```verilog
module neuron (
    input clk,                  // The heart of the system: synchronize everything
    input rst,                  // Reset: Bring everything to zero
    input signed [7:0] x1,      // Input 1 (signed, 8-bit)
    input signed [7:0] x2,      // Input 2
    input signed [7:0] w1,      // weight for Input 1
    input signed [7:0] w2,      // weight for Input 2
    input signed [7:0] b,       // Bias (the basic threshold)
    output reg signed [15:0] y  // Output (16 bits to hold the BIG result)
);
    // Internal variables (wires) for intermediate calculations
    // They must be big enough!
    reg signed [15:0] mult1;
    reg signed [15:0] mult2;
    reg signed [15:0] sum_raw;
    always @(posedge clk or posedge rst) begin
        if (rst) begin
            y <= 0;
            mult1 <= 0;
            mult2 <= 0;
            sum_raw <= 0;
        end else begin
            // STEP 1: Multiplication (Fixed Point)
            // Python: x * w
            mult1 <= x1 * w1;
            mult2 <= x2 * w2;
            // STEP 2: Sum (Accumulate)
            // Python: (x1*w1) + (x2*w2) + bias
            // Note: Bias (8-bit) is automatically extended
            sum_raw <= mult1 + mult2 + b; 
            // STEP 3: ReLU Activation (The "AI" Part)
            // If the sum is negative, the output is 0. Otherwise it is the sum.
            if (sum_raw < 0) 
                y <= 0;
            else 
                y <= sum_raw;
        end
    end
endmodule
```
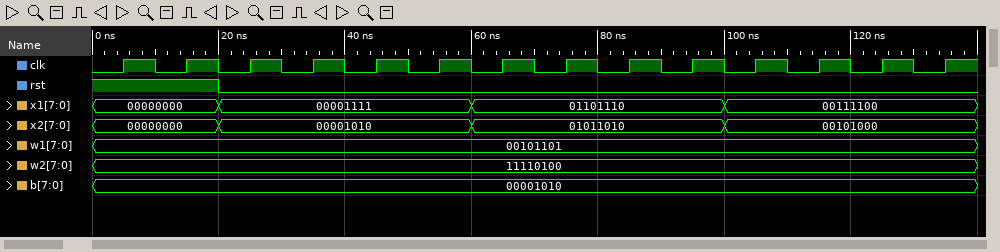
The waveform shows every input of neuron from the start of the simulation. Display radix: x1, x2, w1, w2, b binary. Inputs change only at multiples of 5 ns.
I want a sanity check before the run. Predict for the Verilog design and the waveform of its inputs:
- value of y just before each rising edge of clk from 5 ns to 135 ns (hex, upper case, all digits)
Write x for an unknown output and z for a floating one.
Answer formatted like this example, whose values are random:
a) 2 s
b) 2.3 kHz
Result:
a) 0000, 0000, 0000, 0000, 000A, 0235, 0235, 0235, 0235, 0F28, 0F28, 0F28, 0F28, 08B6
